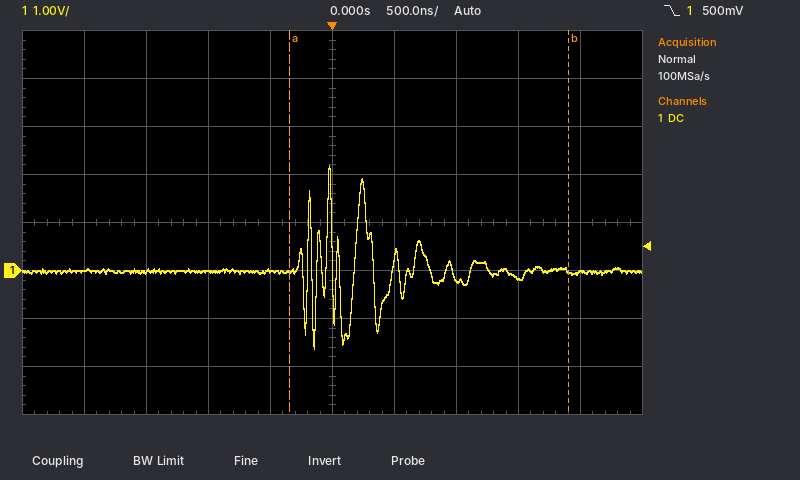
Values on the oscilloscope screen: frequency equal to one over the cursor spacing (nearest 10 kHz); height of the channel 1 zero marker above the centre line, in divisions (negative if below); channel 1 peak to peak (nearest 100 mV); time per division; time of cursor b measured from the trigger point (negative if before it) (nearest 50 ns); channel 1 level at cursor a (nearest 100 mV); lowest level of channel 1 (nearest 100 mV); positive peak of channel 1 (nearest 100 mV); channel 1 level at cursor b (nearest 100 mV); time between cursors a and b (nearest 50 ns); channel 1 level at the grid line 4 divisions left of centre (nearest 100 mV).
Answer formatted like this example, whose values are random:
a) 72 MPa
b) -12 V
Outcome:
a) 440 kHz
b) -1.0 div
c) 3.8 V
d) 500 ns
e) +1.90 µs
f) 0.0 V
g) -1.6 V
h) 2.2 V
i) 0.0 V
j) 2.25 µs
k) 0.0 V
